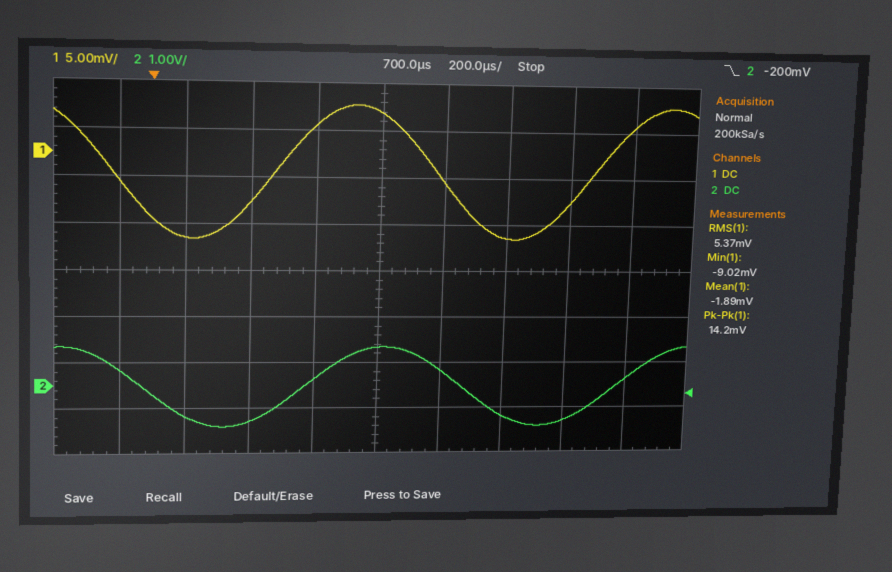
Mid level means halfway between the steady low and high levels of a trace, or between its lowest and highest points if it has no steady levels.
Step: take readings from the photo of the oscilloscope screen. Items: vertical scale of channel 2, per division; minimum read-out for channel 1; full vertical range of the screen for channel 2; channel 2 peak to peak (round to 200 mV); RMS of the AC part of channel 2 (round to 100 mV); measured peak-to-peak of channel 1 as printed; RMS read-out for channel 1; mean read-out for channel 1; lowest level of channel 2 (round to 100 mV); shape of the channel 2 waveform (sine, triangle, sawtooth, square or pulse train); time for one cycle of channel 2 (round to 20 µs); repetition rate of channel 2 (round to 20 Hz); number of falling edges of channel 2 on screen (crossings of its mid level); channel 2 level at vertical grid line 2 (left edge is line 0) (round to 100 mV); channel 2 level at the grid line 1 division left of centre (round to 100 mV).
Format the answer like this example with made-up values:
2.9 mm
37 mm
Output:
1 V
-9.02 mV
8 V
1.8 V
600 mV
14.2 mV
5.37 mV
-1.89 mV
-900 mV
sine
1.00 ms
1.00 kHz
2
-700 mV
100 mV
